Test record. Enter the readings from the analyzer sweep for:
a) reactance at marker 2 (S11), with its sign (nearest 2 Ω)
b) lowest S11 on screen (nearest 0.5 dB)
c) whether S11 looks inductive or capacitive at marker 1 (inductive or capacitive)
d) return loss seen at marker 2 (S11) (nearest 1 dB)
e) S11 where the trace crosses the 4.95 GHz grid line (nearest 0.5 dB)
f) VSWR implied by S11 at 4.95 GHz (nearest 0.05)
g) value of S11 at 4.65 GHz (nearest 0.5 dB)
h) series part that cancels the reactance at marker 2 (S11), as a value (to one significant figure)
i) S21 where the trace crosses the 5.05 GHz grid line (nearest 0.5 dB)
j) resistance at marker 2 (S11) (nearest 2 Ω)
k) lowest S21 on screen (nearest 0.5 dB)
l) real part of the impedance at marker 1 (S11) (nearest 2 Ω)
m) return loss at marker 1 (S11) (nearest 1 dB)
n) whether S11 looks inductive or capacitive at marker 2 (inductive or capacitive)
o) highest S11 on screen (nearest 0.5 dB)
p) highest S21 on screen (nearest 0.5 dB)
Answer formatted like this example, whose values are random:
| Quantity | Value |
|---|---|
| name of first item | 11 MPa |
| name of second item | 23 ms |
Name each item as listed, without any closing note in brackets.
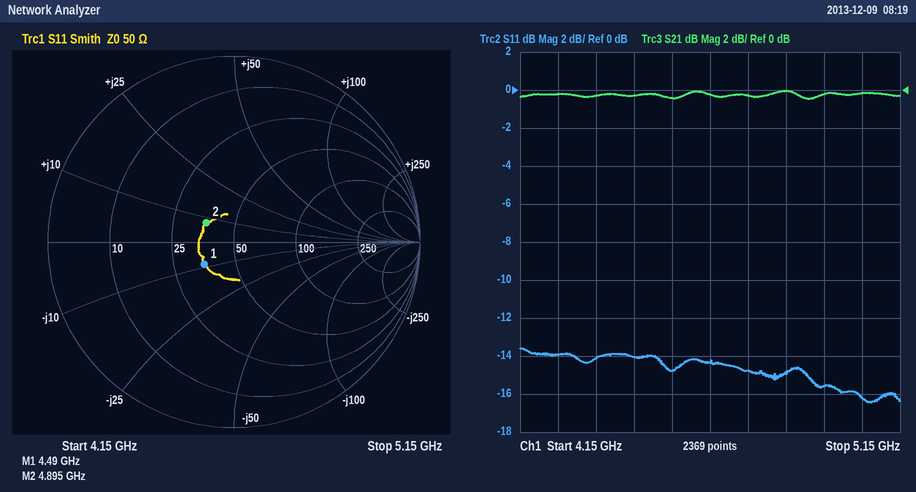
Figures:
| Quantity | Value |
|---|---|
| reactance at marker 2 (S11), with its sign | +8 Ω |
| lowest S11 on screen | -16.5 dB |
| whether S11 looks inductive or capacitive at marker 1 | capacitive |
| return loss seen at marker 2 (S11) | 15 dB |
| S11 where the trace crosses the 4.95 GHz grid line | -15.5 dB |
| VSWR implied by S11 at 4.95 GHz | 1.40 |
| value of S11 at 4.65 GHz | -14.5 dB |
| series part that cancels the reactance at marker 2 (S11), as a value | 4 pF |
| S21 where the trace crosses the 5.05 GHz grid line | 0.0 dB |
| resistance at marker 2 (S11) | 36 Ω |
| lowest S21 on screen | -0.5 dB |
| real part of the impedance at marker 1 (S11) | 36 Ω |
| return loss at marker 1 (S11) | 14 dB |
| whether S11 looks inductive or capacitive at marker 2 | inductive |
| highest S11 on screen | -13.5 dB |
| highest S21 on screen | 0.0 dB |
